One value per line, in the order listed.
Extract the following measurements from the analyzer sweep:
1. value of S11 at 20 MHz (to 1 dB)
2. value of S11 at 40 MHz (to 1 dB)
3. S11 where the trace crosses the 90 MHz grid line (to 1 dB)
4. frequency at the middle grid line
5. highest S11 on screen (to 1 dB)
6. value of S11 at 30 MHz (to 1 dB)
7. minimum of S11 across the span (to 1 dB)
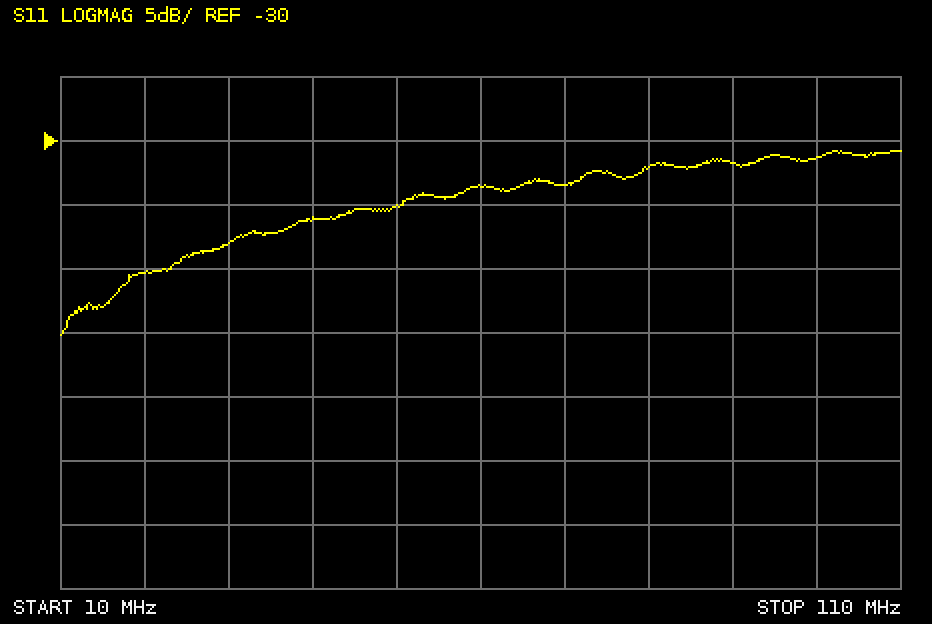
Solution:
-40 dB
-36 dB
-32 dB
60 MHz
-31 dB
-38 dB
-45 dB
